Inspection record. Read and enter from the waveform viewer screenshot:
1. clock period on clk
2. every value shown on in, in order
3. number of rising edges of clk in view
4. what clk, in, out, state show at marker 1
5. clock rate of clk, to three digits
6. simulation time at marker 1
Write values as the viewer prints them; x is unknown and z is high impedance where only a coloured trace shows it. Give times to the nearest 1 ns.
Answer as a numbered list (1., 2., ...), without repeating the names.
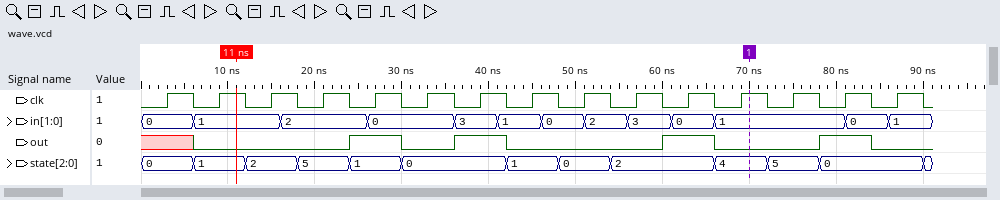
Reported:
1. 6 ns
2. 0, 1, 2, 0, 3, 1, 0, 2, 3, 0, 1, 0, 1
3. 15
4. clk=1, in=1, out=0, state=4
5. 167 MHz
6. 70 ns
